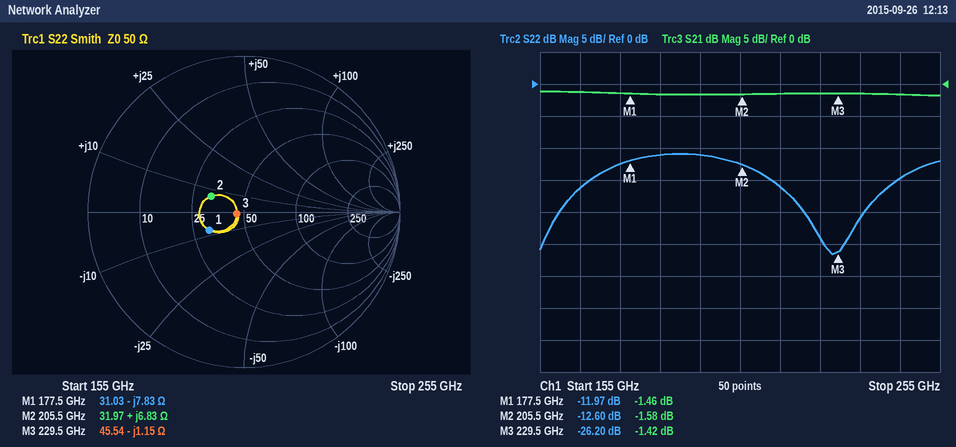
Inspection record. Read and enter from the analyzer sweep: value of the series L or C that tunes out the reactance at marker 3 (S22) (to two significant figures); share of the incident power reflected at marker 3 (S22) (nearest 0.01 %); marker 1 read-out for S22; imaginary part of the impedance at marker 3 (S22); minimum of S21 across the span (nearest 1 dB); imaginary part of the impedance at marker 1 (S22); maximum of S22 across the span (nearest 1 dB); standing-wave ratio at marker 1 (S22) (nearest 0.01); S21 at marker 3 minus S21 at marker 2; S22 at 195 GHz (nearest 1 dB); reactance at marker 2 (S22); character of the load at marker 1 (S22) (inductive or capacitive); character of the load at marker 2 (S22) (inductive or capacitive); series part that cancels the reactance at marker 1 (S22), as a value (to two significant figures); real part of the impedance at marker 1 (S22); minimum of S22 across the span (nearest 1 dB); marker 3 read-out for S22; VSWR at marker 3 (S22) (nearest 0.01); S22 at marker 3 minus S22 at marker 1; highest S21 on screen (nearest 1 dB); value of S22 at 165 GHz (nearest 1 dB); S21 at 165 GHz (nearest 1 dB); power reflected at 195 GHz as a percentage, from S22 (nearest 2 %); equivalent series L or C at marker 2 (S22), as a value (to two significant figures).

800 fH
0.24 %
-11.97 dB
-1.15 Ω
-2 dB
-7.83 Ω
-11 dB
1.67
0.16 dB
-11 dB
+6.83 Ω
capacitive
inductive
7.0 pH
31.03 Ω
-27 dB
-26.20 dB
1.10
-14.23 dB
-1 dB
-16 dB
-1 dB
8 %
5.3 pH
